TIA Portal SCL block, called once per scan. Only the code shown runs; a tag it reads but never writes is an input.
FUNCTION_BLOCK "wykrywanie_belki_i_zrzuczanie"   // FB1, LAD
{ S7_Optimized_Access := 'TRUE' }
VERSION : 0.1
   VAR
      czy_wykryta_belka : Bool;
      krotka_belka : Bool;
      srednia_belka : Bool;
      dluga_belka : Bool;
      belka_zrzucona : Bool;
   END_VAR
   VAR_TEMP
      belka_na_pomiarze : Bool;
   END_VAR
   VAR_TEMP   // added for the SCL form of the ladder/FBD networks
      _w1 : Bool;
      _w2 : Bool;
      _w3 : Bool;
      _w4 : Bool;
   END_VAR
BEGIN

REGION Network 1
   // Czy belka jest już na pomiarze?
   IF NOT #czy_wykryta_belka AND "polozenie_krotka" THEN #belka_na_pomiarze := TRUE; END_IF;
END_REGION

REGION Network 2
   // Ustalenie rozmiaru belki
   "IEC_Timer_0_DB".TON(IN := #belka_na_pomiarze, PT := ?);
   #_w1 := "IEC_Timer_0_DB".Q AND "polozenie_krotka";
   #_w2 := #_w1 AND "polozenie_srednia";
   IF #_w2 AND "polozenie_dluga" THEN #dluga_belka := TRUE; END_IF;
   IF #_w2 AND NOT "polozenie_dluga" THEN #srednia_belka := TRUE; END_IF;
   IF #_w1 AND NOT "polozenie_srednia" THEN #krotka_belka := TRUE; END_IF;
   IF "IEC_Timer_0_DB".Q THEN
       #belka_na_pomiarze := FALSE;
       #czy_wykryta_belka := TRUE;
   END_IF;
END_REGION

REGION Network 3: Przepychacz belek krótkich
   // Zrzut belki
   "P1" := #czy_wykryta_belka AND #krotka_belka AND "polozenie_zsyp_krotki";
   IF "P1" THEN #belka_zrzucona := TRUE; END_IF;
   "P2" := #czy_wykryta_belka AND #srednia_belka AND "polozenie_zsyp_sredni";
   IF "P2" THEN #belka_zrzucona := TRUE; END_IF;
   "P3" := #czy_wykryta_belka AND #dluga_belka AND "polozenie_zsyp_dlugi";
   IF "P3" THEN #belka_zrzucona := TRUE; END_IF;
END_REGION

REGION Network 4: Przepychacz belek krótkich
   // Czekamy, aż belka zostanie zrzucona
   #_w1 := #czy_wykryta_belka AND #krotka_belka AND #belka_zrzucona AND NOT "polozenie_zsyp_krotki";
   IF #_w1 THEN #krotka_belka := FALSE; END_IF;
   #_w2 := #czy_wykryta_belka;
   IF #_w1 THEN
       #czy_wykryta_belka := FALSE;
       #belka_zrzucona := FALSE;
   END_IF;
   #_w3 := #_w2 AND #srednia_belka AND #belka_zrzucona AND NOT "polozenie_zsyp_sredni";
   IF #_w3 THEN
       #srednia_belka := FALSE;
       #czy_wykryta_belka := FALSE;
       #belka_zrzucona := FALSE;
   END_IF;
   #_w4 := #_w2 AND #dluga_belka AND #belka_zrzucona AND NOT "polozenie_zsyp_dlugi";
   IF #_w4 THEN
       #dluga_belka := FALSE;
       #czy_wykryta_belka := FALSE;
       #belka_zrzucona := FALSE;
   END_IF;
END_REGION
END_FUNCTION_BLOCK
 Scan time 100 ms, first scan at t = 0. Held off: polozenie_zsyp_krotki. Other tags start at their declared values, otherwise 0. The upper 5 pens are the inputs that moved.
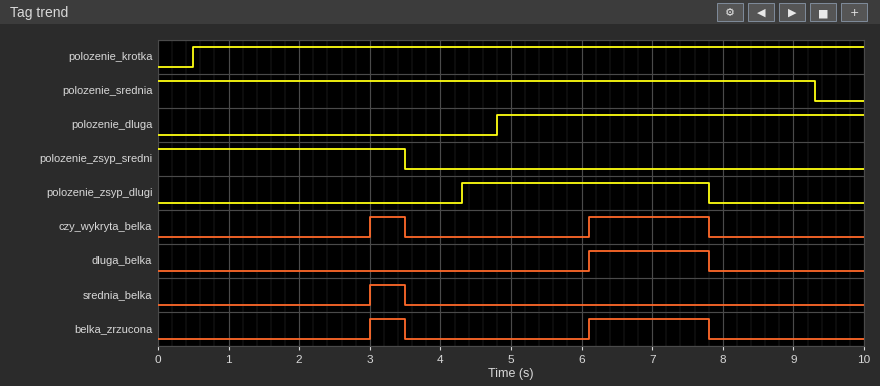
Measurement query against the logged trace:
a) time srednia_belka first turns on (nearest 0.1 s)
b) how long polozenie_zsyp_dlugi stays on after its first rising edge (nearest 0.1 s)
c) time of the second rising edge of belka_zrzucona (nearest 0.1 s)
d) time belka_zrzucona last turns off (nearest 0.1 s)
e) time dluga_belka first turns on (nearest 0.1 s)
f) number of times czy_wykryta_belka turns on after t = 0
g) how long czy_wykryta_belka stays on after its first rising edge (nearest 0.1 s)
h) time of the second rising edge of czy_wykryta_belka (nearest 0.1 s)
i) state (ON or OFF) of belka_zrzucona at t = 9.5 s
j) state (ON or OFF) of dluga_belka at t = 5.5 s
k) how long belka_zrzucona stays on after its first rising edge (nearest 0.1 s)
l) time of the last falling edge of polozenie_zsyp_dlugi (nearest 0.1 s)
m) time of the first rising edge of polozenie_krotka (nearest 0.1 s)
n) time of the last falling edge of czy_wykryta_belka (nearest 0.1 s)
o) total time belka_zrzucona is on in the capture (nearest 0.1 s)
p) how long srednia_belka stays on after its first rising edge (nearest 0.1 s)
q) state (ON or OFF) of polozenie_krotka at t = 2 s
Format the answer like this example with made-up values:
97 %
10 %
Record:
3.0 s
3.5 s
6.1 s
7.8 s
6.1 s
2
0.5 s
6.1 s
OFF
OFF
0.5 s
7.8 s
0.5 s
7.8 s
2.2 s
0.5 s
ON
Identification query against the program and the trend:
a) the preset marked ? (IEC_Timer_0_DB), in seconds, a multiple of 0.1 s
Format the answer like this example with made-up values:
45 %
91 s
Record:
2.5 s
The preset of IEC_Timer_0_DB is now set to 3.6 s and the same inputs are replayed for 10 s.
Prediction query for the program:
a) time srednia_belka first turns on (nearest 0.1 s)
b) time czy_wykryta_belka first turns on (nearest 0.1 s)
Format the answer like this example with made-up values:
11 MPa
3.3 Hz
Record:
4.1 s
4.1 s
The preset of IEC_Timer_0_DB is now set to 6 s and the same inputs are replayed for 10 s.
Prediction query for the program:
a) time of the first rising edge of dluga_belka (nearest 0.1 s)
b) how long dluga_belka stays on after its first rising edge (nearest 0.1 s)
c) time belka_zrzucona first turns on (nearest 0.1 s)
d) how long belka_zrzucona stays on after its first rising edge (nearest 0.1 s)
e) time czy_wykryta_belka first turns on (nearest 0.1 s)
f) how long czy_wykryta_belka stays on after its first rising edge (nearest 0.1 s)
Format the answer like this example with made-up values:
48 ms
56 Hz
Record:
6.5 s
1.3 s
6.5 s
1.3 s
6.5 s
1.3 s
